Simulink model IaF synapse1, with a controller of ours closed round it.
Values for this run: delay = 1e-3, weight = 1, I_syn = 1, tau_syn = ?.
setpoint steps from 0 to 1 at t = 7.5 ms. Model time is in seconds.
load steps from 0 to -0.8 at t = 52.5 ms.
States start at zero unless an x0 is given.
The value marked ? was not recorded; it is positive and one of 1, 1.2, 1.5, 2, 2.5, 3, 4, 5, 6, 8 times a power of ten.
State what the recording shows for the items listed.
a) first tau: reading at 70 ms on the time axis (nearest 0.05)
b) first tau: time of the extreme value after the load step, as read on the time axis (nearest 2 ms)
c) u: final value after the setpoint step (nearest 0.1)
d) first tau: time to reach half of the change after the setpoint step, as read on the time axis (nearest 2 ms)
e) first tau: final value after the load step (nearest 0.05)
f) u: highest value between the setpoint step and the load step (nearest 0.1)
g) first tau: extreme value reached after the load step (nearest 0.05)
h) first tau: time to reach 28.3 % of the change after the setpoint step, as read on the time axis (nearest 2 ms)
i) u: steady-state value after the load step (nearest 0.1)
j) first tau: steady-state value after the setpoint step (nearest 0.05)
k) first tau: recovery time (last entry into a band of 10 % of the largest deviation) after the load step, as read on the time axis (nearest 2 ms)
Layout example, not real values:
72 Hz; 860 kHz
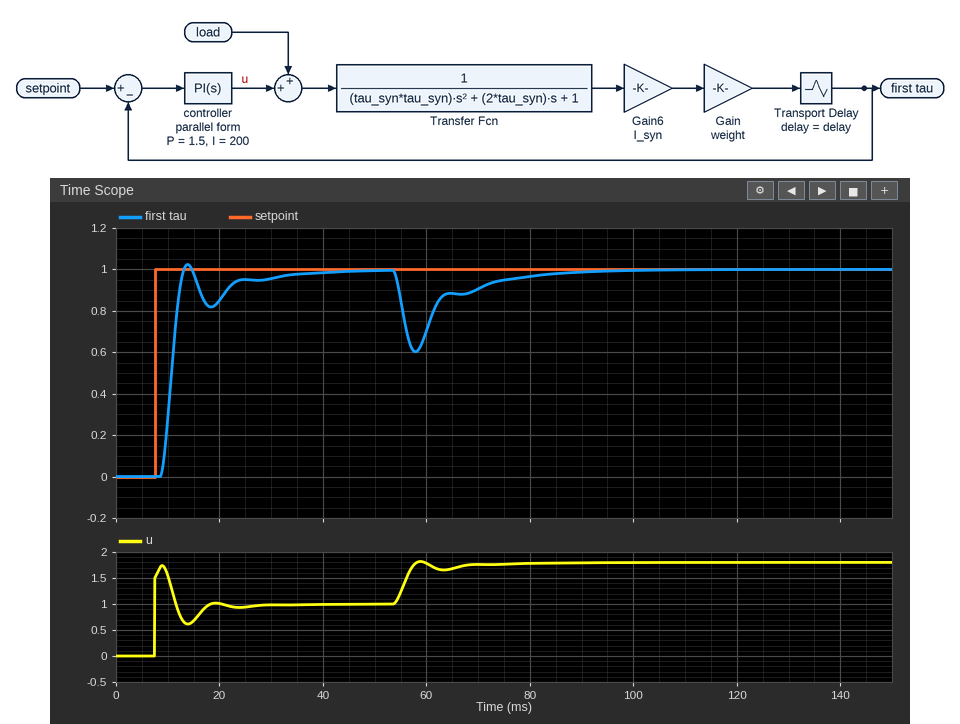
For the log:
0.90; 58 ms; 1.0; 10 ms; 1.00; 1.7; 0.60; 10 ms; 1.8; 1.00; 78 ms
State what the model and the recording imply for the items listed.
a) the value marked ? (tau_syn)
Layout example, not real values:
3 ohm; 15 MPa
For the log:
0.002
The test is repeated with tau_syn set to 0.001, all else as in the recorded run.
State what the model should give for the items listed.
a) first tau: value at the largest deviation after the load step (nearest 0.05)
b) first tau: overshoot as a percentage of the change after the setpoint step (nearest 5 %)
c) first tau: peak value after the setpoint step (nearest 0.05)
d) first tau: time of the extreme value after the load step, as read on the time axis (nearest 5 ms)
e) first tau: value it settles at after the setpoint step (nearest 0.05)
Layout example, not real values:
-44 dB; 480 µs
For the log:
0.50; 10 %; 1.10; 55 ms; 1.00
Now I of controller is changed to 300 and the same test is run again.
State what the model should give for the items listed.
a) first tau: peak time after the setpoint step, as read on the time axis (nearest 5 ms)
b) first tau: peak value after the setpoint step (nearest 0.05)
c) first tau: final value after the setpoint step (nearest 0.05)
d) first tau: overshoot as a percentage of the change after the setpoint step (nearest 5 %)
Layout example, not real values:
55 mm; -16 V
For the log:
15 ms; 1.15; 1.00; 15 %
